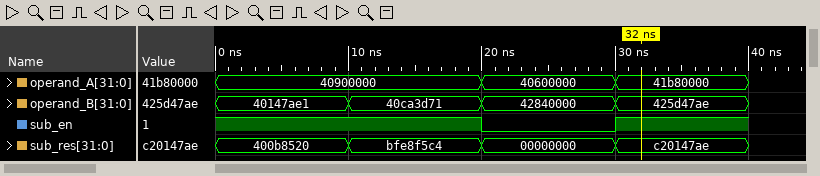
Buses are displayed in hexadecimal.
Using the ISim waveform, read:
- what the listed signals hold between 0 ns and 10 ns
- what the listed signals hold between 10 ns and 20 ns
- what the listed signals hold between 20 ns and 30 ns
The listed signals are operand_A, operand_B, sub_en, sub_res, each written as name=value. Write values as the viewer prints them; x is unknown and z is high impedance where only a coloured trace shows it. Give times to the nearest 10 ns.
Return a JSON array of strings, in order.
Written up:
["operand_A=40900000, operand_B=40147ae1, sub_en=1, sub_res=400b8520", "operand_A=40900000, operand_B=40ca3d71, sub_en=1, sub_res=bfe8f5c4", "operand_A=40600000, operand_B=42840000, sub_en=0, sub_res=00000000"]
